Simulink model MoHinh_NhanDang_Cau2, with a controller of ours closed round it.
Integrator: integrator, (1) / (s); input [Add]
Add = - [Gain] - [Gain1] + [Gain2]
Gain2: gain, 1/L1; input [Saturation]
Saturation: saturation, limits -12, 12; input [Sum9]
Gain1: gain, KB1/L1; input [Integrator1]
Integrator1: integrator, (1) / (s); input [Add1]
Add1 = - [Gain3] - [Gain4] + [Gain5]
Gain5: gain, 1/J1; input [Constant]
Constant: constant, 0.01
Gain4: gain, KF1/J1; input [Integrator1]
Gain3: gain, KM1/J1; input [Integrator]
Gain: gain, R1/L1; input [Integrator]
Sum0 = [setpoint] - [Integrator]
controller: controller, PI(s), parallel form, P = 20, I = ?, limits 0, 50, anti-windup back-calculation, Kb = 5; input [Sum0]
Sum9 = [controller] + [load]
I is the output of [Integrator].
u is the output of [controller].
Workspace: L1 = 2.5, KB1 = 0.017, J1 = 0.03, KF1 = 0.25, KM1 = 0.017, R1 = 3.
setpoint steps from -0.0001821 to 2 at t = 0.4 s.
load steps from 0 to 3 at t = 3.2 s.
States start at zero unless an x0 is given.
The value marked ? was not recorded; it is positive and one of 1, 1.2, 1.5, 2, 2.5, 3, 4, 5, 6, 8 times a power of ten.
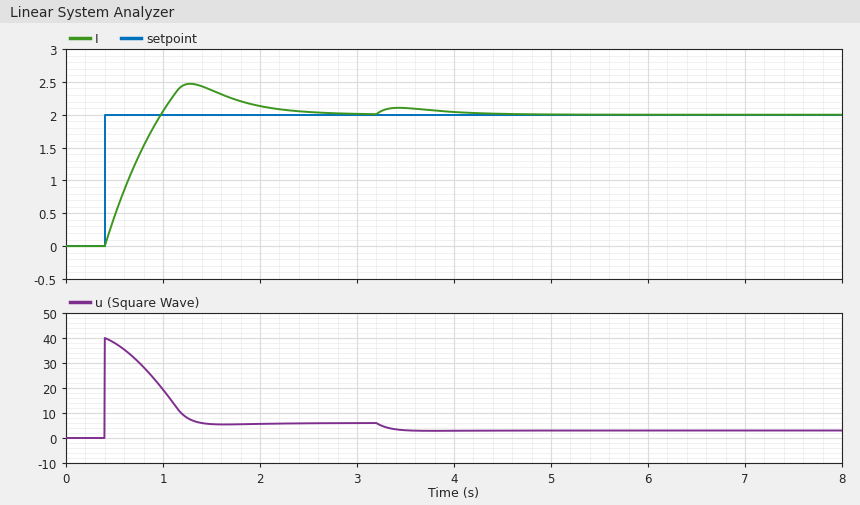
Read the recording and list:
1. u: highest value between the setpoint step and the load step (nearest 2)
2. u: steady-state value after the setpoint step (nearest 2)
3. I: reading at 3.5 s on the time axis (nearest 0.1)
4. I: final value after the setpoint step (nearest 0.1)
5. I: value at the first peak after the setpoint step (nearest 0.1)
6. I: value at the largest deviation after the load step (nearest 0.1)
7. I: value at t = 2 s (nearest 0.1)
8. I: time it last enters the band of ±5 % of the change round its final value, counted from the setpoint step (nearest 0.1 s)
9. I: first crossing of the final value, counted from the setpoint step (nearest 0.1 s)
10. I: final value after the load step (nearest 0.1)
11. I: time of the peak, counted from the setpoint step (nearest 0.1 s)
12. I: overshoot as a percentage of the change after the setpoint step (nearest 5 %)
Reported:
40
6
2.1
2.0
2.5
2.1
2.1
1.7 s
0.6 s
2.0
0.9 s
25 %
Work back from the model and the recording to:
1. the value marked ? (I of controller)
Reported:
40
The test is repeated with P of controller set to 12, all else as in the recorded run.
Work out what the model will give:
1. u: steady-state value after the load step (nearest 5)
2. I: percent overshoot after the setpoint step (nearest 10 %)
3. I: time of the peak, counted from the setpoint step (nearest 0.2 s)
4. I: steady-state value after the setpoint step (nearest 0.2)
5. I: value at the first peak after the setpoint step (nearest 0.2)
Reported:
5
30 %
1.0 s
2.0
2.6
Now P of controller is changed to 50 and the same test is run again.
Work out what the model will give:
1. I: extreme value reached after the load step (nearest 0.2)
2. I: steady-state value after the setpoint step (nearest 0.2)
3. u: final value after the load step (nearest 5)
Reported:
2.0
2.0
5
